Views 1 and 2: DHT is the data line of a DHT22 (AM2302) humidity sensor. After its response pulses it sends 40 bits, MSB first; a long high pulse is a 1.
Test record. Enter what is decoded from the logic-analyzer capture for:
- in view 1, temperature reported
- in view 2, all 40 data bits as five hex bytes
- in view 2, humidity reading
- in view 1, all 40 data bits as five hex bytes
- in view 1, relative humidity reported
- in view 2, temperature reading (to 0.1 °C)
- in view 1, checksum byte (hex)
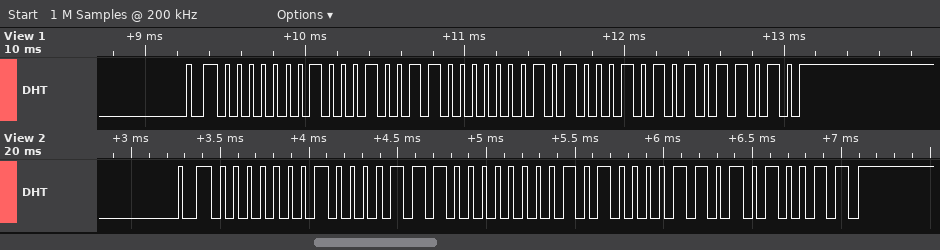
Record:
32.5 °C
01 0E 01 43 53
27.0 %
01 13 01 45 5A
27.5 %
32.3 °C
0x5A
